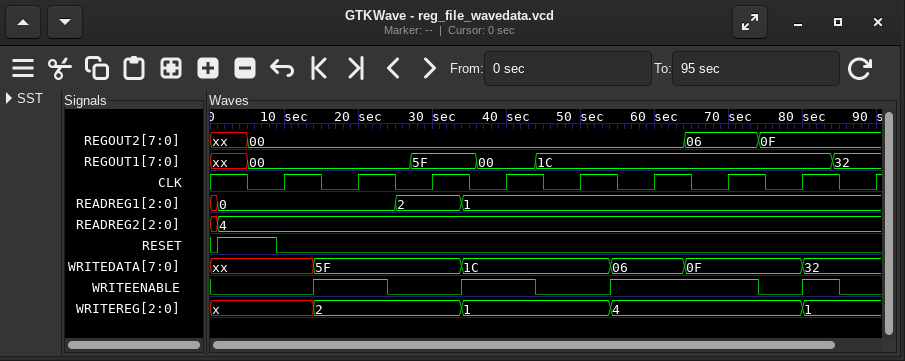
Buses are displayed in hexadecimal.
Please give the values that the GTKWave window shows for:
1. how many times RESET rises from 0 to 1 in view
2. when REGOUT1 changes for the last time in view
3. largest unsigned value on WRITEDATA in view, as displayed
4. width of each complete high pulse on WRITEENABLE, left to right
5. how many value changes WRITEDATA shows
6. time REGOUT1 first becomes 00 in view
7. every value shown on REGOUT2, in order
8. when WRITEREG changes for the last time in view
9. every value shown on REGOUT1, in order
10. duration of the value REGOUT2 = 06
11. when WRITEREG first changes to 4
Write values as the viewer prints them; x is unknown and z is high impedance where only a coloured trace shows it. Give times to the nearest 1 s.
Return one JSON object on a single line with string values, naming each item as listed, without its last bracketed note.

{"how many times RESET rises from 0 to 1 in view": "1", "when REGOUT1 changes for the last time in view": "84 s", "largest unsigned value on WRITEDATA in view, as displayed": "5F", "width of each complete high pulse on WRITEENABLE, left to right": "10 s, 10 s, 20 s, 5 s", "how many value changes WRITEDATA shows": "5", "time REGOUT1 first becomes 00 in view": "5 s", "every value shown on REGOUT2, in order": "xx, 00, 06, 0F", "when WRITEREG changes for the last time in view": "80 s", "every value shown on REGOUT1, in order": "xx, 00, 5F, 00, 1C, 32", "duration of the value REGOUT2 = 06": "10 s", "when WRITEREG first changes to 4": "54 s"}
